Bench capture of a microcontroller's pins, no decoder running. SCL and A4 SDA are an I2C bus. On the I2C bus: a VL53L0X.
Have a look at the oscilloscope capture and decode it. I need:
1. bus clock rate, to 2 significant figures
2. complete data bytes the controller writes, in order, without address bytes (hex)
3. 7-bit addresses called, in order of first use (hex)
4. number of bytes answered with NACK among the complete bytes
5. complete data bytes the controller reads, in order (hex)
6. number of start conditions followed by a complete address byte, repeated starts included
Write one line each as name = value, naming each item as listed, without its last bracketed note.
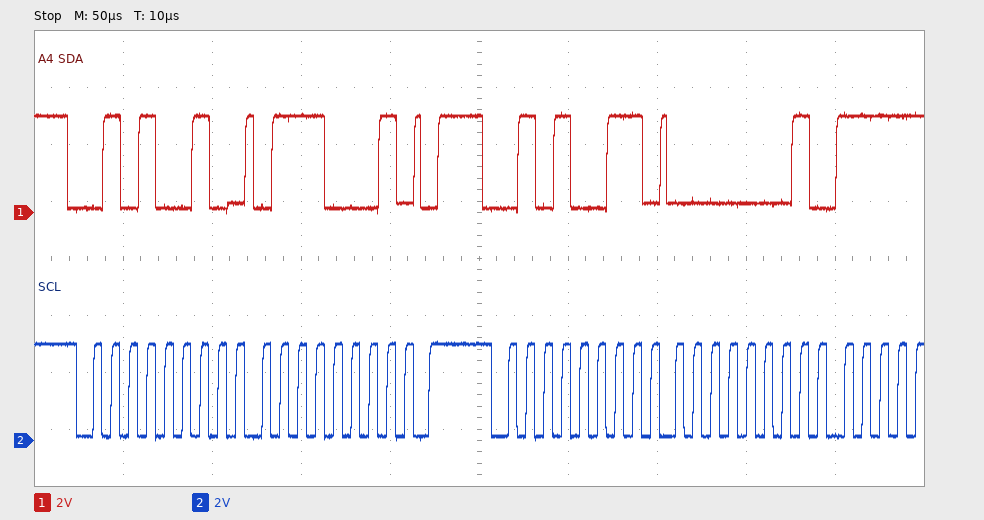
bus clock rate, to 2 significant figures = 100 kHz
complete data bytes the controller writes, in order, without address bytes = 71
7-bit addresses called, in order of first use = 0x29
number of bytes answered with NACK among the complete bytes = 0
complete data bytes the controller reads, in order = 01
number of start conditions followed by a complete address byte, repeated starts included = 2
